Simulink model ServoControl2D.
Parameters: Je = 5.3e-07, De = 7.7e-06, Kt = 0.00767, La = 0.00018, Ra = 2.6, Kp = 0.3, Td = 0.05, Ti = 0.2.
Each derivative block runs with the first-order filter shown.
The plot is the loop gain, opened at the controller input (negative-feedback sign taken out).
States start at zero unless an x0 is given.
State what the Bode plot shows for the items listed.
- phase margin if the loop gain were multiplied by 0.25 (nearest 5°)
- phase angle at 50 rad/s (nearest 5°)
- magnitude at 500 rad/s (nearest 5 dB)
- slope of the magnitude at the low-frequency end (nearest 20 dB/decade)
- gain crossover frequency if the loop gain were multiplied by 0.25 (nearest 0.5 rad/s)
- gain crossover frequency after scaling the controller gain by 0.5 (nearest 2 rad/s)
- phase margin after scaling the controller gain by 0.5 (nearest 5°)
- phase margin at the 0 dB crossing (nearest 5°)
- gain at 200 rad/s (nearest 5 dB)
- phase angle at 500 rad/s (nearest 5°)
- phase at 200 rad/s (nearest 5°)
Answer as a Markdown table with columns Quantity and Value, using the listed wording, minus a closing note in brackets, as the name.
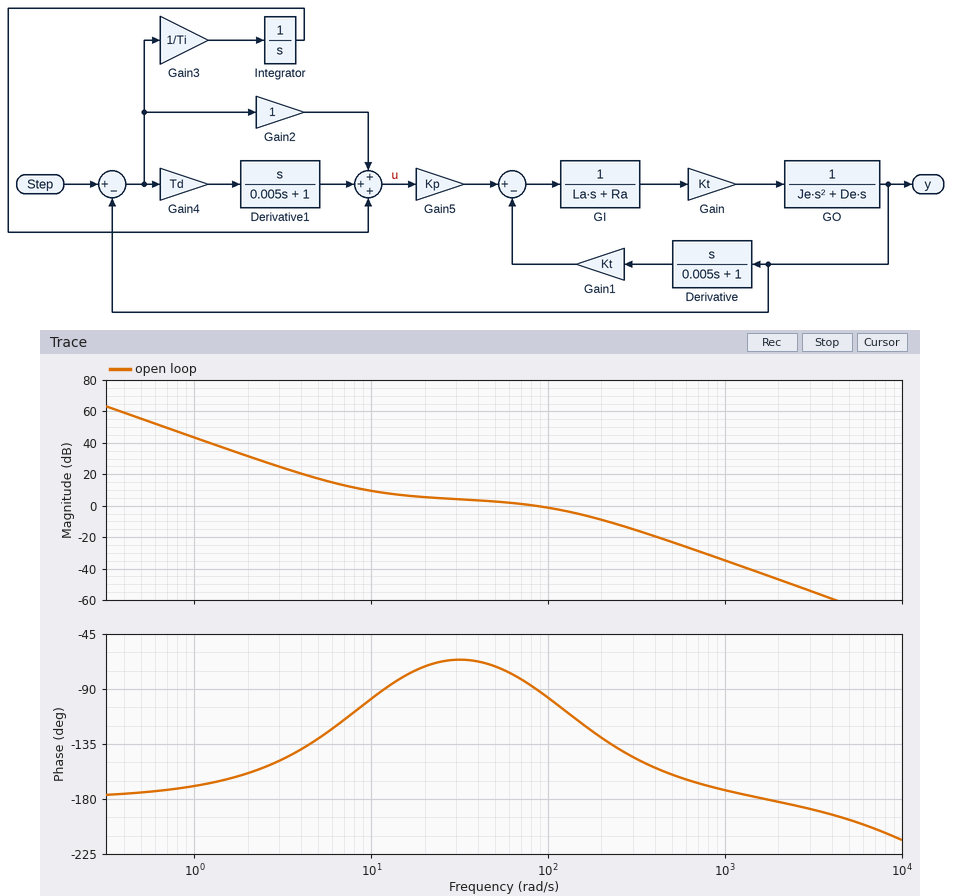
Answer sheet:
| Quantity | Value |
|---|---|
| phase margin if the loop gain were multiplied by 0.25 | 70° |
| phase angle at 50 rad/s | -70° |
| magnitude at 500 rad/s | -25 dB |
| slope of the magnitude at the low-frequency end | -40 dB/decade |
| gain crossover frequency if the loop gain were multiplied by 0.25 | 7.5 rad/s |
| gain crossover frequency after scaling the controller gain by 0.5 | 18 rad/s |
| phase margin after scaling the controller gain by 0.5 | 105° |
| phase margin at the 0 dB crossing | 90° |
| gain at 200 rad/s | -10 dB |
| phase angle at 500 rad/s | -160° |
| phase at 200 rad/s | -130° |
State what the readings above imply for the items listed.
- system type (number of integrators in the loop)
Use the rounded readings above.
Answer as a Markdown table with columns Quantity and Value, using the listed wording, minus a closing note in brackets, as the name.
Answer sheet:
| Quantity | Value |
|---|---|
| system type | 2 |
